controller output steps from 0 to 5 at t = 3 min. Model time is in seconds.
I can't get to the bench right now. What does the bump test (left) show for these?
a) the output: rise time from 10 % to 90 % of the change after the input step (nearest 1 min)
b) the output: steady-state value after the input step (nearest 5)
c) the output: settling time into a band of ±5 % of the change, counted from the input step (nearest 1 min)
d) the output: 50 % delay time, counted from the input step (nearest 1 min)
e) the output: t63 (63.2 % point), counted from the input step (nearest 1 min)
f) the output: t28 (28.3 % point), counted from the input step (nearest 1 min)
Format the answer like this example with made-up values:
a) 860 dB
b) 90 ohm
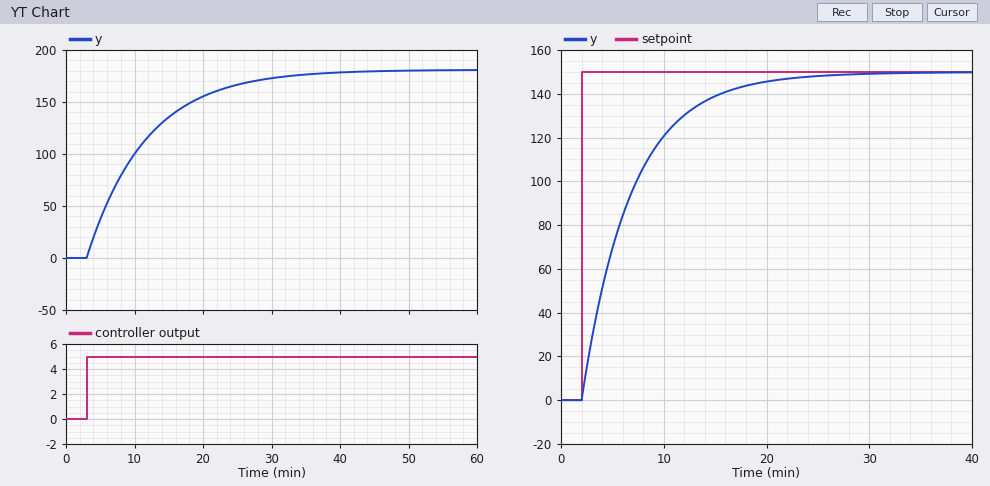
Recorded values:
a) 19 min
b) 180
c) 26 min
d) 6 min
e) 9 min
f) 3 min
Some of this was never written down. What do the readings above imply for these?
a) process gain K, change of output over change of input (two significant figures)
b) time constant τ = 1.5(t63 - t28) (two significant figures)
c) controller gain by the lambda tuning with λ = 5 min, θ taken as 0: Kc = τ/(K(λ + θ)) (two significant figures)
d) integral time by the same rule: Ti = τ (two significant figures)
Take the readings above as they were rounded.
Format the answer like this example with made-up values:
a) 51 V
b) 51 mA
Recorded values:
a) 36
b) 9.0 min
c) 0.050
d) 9.0 min
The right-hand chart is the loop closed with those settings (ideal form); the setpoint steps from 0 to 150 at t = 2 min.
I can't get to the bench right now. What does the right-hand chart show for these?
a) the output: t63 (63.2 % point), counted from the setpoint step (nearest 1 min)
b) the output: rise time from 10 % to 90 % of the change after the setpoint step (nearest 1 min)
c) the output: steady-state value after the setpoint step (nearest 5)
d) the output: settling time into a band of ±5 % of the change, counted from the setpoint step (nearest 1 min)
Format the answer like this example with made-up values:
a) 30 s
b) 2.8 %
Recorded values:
a) 5 min
b) 11 min
c) 150
d) 15 min
